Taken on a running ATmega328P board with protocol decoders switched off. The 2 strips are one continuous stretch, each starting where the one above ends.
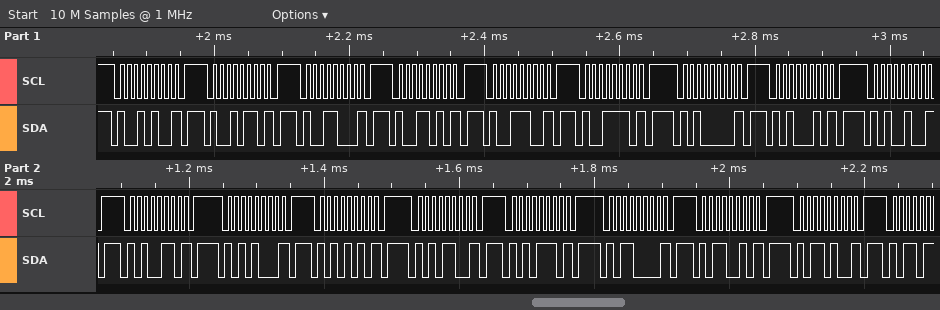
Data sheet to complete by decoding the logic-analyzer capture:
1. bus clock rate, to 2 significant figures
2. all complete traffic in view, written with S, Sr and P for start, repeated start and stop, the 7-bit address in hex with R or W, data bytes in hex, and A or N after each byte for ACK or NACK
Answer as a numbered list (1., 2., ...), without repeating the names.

1. 100 kHz
2. S 4AW N P S 4BW N P S 4CW N P S 4DW N P S 4EW N P S 4FW N P S 50W N P S 51W N P S 52W N P S 53W N P S 54W N P S 55W N P S 56W N P S 57W N P S 58W N P S 59W N P S 5AW N P
